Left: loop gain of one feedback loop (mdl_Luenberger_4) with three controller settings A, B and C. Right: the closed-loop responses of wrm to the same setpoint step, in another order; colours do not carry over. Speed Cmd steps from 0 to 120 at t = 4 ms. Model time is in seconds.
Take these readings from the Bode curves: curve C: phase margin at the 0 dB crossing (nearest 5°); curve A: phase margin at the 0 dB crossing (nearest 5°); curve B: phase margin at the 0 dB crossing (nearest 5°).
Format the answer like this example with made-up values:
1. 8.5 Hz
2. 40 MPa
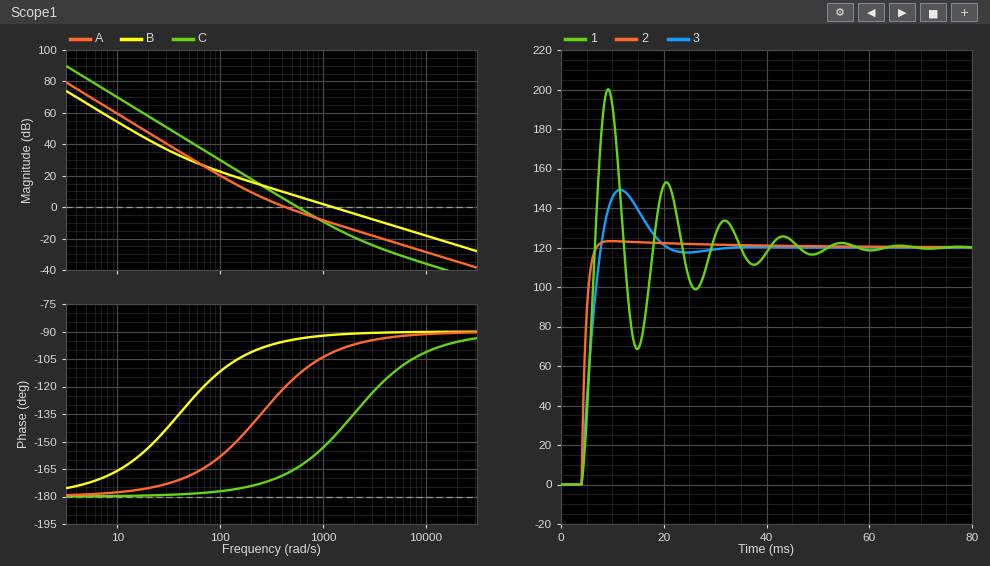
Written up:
1. 15°
2. 60°
3. 90°
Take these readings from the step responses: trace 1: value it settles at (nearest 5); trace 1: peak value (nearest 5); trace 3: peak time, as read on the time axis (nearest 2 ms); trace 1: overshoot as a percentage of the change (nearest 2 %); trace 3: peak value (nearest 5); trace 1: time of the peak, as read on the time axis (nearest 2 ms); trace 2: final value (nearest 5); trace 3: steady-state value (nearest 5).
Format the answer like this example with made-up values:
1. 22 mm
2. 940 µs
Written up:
1. 120
2. 200
3. 12 ms
4. 66 %
5. 150
6. 10 ms
7. 120
8. 120
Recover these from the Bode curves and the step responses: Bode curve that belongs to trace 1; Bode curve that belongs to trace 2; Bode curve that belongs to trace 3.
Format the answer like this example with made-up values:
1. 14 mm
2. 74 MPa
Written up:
1. C
2. B
3. A
